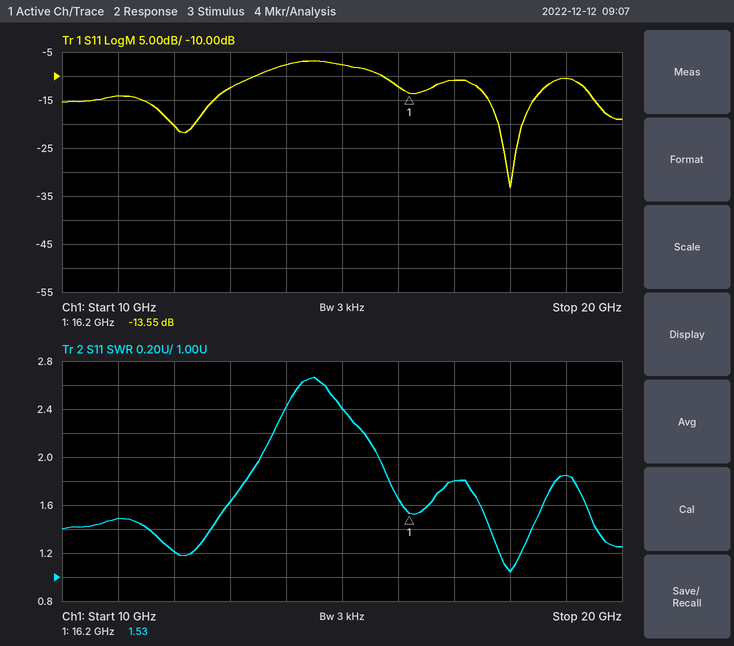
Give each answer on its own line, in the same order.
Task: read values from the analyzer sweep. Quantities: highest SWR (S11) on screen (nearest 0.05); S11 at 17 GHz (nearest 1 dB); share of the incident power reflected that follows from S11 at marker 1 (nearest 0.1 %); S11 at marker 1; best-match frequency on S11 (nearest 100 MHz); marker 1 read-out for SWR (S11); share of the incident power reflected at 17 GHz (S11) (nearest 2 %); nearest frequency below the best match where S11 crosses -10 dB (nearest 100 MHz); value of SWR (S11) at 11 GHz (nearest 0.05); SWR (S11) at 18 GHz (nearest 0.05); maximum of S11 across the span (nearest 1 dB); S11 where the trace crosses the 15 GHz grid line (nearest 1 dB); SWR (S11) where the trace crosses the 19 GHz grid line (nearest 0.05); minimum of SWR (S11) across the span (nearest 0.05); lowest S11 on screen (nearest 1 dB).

2.65
-11 dB
4.4 %
-13.55 dB
18.0 GHz
1.53
8 %
15.7 GHz
1.50
1.05
-7 dB
-8 dB
1.85
1.05
-33 dB
